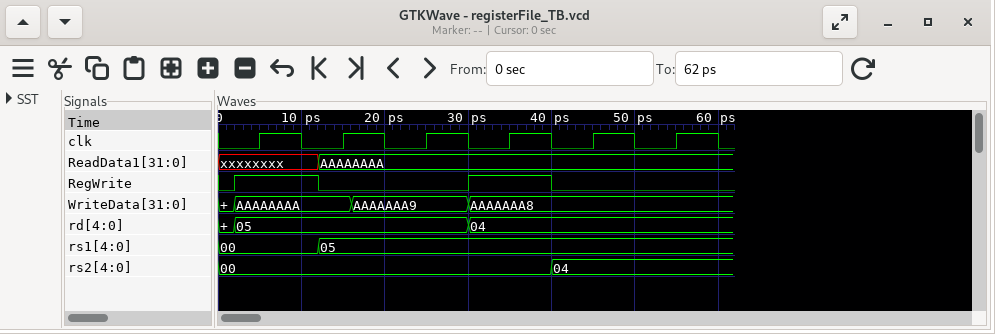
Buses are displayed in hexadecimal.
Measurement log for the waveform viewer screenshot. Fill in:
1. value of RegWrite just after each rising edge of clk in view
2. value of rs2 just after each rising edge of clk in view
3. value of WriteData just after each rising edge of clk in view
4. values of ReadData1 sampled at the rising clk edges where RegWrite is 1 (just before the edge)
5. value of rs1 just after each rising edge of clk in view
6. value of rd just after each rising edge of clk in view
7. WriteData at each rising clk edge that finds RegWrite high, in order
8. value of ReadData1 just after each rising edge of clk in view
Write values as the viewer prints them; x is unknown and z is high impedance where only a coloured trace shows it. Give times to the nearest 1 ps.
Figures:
1 0 0 1 0 0
00, 00, 00, 00, 04, 04
AAAAAAAA, AAAAAAAA, AAAAAAA9, AAAAAAA8, AAAAAAA8, AAAAAAA8
xxxxxxxx, AAAAAAAA
00, 05, 05, 05, 05, 05
05, 05, 05, 04, 04, 04
AAAAAAAA, AAAAAAA8
xxxxxxxx, AAAAAAAA, AAAAAAAA, AAAAAAAA, AAAAAAAA, AAAAAAAA
